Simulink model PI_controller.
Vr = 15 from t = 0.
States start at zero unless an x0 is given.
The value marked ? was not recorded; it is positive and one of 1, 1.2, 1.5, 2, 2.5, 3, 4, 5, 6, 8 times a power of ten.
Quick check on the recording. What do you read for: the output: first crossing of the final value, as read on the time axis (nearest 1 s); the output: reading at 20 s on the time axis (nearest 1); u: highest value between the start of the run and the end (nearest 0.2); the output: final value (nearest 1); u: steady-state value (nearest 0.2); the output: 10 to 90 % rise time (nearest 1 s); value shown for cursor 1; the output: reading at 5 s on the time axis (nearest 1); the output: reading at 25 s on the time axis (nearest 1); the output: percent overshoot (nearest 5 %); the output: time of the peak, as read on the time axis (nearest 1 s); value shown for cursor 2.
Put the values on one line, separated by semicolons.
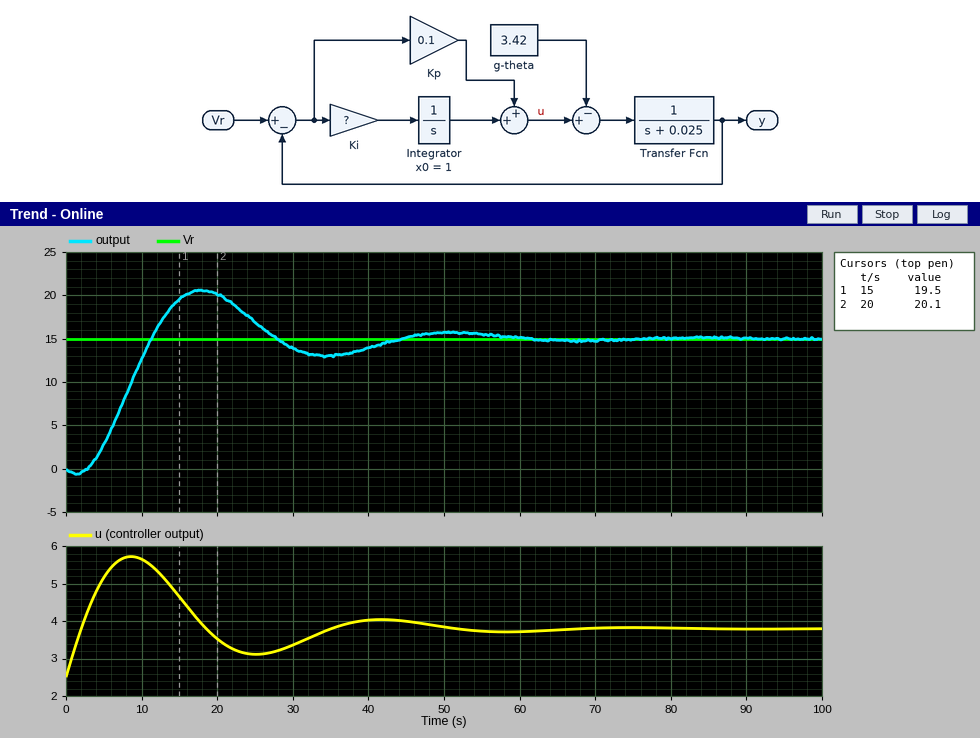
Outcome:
11 s; 20; 5.8; 15; 3.8; 6 s; 19.5; 3; 17; 35 %; 18 s; 20.1
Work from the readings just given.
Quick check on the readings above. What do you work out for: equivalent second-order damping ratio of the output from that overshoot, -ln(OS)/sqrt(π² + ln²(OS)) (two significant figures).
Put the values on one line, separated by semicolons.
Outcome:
0.32
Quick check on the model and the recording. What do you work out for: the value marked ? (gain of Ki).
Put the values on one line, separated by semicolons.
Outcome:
0.04
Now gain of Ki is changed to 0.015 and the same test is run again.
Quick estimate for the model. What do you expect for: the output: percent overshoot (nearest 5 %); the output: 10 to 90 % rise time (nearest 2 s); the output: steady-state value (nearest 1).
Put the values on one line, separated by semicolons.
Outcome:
15 %; 12 s; 15
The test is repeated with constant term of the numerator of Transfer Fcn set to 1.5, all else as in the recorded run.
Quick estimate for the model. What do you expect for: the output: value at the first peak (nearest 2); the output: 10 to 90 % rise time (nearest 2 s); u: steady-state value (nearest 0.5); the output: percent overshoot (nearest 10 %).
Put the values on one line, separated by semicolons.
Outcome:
20; 6 s; 3.5; 30 %
